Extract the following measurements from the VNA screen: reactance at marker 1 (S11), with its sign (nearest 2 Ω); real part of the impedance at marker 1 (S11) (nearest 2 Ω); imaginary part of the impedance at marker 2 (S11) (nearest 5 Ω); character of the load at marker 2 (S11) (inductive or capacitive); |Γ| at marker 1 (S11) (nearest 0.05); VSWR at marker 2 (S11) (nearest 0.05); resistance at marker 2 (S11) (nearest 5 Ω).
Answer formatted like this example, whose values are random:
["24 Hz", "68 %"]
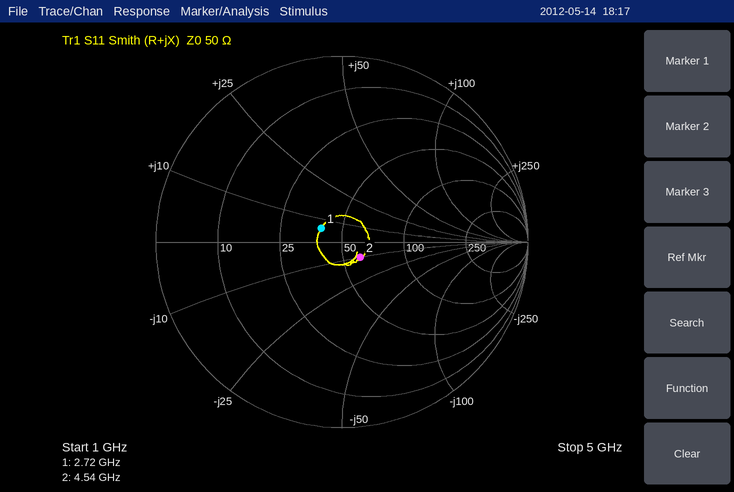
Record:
["+6 Ω", "40 Ω", "-10 Ω", "capacitive", "0.15", "1.30", "60 Ω"]
